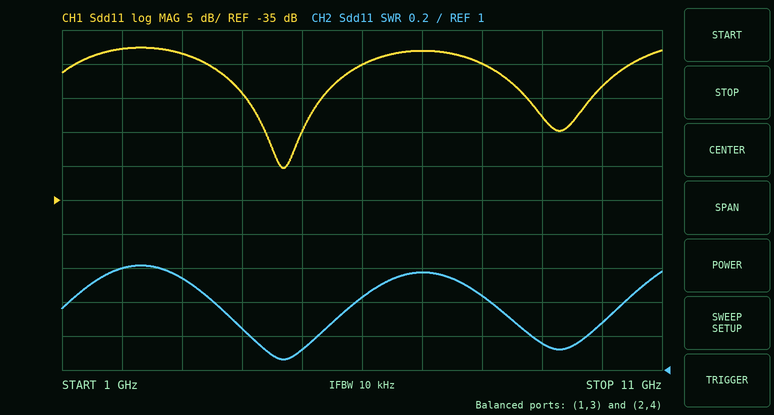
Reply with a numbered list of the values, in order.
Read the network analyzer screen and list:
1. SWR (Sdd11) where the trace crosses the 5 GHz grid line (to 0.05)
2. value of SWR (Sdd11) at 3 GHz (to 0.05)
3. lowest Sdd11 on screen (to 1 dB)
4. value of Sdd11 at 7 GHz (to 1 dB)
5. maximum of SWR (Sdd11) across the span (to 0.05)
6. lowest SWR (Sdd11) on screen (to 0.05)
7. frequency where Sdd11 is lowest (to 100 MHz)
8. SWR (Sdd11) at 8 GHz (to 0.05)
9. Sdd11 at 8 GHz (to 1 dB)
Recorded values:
1. 1.10
2. 1.55
3. -30 dB
4. -13 dB
5. 1.60
6. 1.05
7. 4.7 GHz
8. 1.45
9. -15 dB
